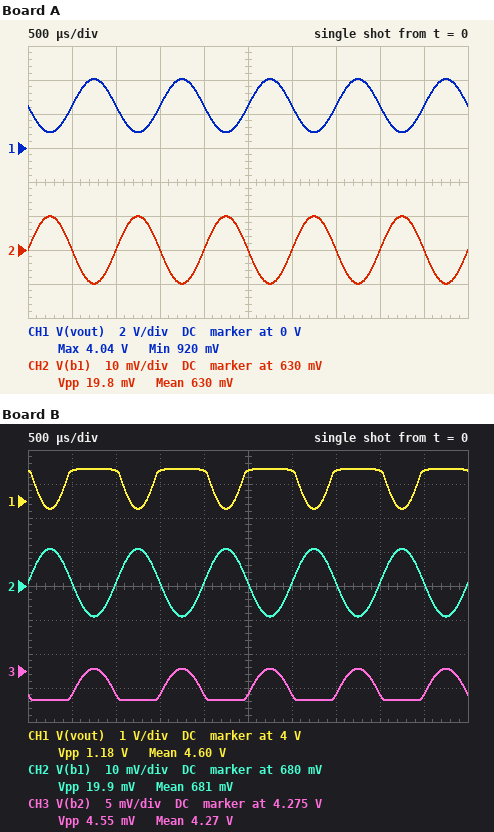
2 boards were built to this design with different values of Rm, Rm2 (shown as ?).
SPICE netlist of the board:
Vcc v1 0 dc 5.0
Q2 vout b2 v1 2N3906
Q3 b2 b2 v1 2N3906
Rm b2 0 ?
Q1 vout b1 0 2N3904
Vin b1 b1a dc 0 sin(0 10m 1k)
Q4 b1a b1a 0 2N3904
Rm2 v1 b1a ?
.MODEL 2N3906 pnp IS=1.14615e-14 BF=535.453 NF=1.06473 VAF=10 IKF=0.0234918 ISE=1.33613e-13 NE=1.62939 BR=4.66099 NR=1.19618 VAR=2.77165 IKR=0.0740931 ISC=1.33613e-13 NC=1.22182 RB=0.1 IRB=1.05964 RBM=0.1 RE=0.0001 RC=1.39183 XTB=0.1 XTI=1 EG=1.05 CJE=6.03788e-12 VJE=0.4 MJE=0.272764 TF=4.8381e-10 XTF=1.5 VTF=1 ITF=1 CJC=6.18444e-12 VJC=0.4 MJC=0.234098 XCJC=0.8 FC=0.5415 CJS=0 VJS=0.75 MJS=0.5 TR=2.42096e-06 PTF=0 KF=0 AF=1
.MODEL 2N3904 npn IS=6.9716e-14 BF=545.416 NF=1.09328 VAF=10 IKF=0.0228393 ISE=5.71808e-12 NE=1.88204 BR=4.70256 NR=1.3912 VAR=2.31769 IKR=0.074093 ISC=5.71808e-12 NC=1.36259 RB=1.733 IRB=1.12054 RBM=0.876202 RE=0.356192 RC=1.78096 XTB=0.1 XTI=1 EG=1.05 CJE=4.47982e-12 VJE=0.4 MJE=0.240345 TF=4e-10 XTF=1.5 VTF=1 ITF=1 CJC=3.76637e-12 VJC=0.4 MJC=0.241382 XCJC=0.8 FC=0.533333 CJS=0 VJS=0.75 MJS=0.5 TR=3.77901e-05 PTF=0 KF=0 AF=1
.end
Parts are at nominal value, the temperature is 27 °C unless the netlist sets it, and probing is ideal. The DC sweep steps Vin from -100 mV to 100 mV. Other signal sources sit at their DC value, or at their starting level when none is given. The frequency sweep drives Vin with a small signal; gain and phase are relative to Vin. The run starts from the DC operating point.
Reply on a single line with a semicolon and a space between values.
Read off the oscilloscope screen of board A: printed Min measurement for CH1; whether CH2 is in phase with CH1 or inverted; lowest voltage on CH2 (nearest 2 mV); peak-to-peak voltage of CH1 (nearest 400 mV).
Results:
920 mV; inverted; 620 mV; 3.2 V
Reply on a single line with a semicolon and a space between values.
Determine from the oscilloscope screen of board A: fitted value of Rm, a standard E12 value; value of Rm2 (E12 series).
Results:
18 kΩ; 18 kΩ
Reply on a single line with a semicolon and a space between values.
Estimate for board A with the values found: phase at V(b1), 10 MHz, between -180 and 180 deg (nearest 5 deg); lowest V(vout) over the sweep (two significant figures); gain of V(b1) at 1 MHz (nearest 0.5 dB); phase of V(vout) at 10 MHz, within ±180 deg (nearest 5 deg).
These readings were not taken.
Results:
-5 deg; 45 mV; -1.5 dB; 95 deg
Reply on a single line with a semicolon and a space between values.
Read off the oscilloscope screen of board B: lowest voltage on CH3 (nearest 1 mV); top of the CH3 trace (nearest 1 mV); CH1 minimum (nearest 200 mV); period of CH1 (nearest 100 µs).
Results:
4.271 V; 4.275 V; 3.8 V; 1.0 ms
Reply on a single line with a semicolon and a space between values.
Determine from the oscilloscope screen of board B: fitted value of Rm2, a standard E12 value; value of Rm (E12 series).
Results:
3.3 kΩ; 1.8 kΩ
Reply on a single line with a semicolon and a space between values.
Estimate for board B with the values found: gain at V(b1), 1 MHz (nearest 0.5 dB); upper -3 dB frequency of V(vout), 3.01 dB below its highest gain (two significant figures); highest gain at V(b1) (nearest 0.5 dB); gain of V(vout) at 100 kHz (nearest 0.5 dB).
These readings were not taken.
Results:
0 dB; 580 kHz; 0 dB; 24.0 dB
